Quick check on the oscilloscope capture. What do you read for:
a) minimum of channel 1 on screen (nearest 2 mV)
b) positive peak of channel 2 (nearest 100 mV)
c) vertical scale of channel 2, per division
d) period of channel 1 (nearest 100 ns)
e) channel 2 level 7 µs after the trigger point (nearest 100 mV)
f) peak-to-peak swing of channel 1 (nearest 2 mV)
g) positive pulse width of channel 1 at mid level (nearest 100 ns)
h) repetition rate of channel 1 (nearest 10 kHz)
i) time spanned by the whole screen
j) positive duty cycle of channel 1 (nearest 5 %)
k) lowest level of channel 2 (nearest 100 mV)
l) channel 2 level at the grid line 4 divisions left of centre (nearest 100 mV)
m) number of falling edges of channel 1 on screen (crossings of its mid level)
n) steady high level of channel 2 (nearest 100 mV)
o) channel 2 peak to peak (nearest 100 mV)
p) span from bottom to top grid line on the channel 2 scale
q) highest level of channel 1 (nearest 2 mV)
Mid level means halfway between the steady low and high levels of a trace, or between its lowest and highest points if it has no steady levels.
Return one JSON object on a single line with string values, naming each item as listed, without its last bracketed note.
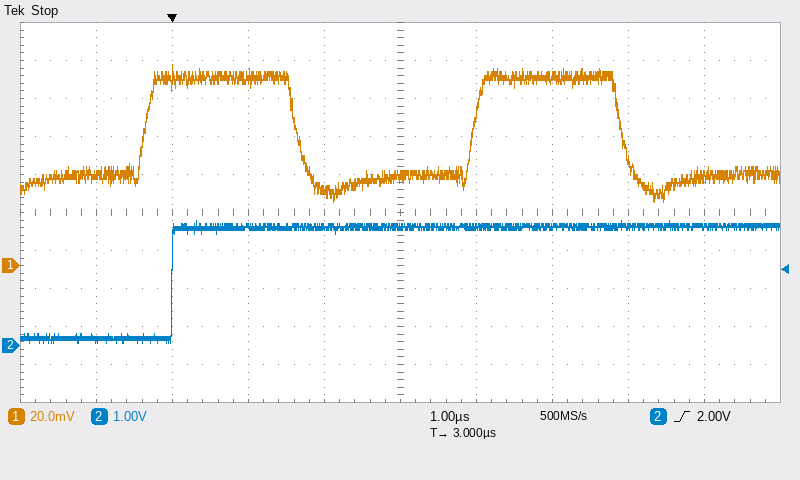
{"minimum of channel 1 on screen": "34 mV", "positive peak of channel 2": "3.3 V", "vertical scale of channel 2, per division": "1 V", "period of channel 1": "4.3 µs", "channel 2 level 7 µs after the trigger point": "3.1 V", "peak-to-peak swing of channel 1": "72 mV", "positive pulse width of channel 1 at mid level": "2.0 µs", "repetition rate of channel 1": "230 kHz", "time spanned by the whole screen": "10 µs", "positive duty cycle of channel 1": "45 %", "lowest level of channel 2": "100 mV", "channel 2 level at the grid line 4 divisions left of centre": "200 mV", "number of falling edges of channel 1 on screen": "2", "steady high level of channel 2": "3.1 V", "channel 2 peak to peak": "3.2 V", "span from bottom to top grid line on the channel 2 scale": "10 V", "highest level of channel 1": "106 mV"}
